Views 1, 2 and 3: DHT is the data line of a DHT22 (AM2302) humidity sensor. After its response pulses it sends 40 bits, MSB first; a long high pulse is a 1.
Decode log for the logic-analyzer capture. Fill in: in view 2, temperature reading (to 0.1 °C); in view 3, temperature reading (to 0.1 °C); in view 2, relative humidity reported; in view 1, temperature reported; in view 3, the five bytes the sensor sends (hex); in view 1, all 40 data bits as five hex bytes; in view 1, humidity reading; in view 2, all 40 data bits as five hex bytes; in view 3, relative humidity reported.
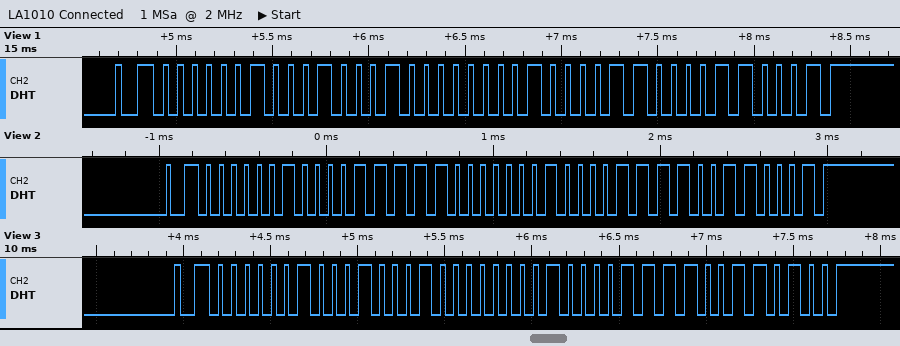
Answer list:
27.1 °C
27.1 °C
54.3 %
26.8 °C
02 22 01 0F 34
02 22 01 0C 31
54.6 %
02 1F 01 0F 31
54.6 %
